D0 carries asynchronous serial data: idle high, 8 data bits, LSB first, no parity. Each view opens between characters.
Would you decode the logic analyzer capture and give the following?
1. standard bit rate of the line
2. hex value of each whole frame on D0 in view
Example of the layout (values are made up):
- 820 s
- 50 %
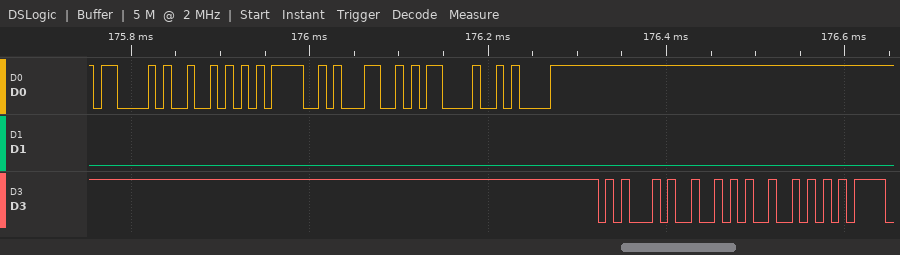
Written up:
- 115200 baud
- 43, 52, 3D, 31, 0D, 0A
